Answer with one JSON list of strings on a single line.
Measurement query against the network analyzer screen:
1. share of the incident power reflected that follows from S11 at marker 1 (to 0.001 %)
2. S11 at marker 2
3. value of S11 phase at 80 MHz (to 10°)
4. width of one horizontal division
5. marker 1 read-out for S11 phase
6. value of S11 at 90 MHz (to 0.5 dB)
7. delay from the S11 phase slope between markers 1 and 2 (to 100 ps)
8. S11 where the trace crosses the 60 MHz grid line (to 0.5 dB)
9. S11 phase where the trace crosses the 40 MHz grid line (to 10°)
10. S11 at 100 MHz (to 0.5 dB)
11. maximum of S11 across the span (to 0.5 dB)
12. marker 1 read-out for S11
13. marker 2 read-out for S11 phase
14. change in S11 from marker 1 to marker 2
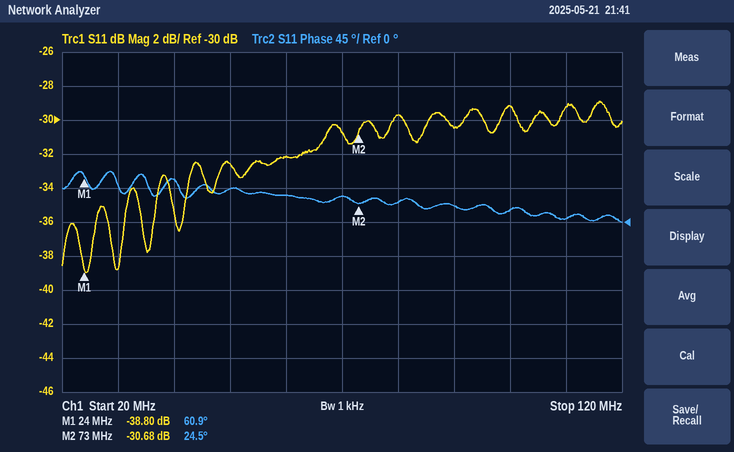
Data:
["0.013 %", "-30.68 dB", "30°", "10 MHz", "60.9°", "-30.5 dB", "2.1 ns", "-32.0 dB", "60°", "-29.0 dB", "-29.0 dB", "-38.80 dB", "24.5°", "8.12 dB"]
